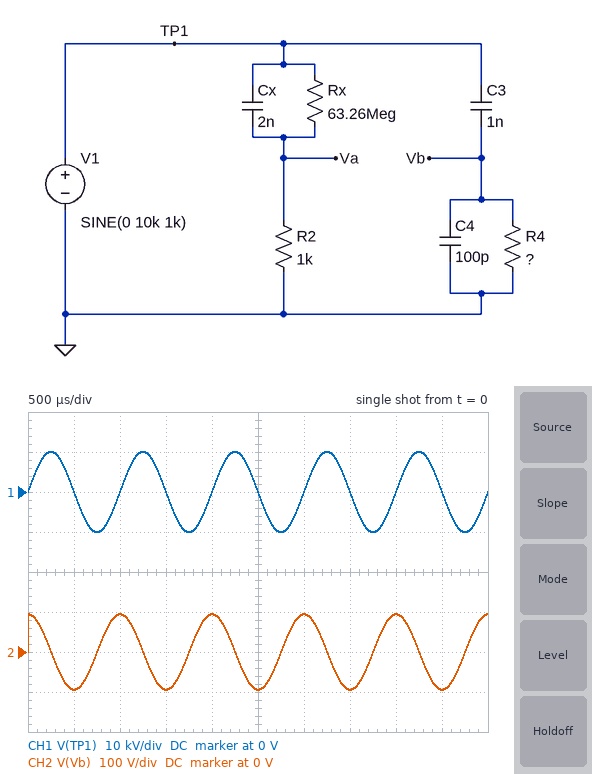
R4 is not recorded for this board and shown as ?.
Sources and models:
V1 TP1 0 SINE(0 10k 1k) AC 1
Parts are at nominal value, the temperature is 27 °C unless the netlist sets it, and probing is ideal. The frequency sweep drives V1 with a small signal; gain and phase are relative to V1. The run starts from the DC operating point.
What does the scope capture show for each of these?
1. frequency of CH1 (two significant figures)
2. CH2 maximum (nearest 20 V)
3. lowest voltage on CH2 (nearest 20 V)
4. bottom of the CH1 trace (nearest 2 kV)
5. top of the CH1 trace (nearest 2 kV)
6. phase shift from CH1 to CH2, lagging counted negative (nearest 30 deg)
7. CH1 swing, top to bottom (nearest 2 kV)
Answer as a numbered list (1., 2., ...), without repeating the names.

1. 1.0 kHz
2. 100 V
3. -100 V
4. -10 kV
5. 10 kV
6. 90 deg
7. 20 kV
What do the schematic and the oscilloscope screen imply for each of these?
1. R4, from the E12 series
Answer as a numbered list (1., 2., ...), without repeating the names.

1. 1.5 kΩ
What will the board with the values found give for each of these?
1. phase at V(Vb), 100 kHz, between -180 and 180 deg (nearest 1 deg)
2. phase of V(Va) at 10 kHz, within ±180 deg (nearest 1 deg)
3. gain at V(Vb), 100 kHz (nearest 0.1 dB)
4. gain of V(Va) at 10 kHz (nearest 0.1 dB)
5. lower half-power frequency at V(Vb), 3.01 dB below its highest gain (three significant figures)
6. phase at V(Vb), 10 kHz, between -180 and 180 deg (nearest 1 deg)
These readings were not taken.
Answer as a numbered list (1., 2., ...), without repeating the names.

1. 44 deg
2. 83 deg
3. -3.7 dB
4. -18.1 dB
5. 96.5 kHz
6. 84 deg
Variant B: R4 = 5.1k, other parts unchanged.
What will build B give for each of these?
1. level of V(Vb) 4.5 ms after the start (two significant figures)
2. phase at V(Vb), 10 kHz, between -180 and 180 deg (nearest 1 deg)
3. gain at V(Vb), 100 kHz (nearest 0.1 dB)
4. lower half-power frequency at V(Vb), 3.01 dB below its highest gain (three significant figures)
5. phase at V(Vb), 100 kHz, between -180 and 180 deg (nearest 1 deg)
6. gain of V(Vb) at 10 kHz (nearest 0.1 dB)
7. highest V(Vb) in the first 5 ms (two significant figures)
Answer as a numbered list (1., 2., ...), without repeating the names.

1. -320 V
2. 71 deg
3. -1.2 dB
4. 28.4 kHz
5. 16 deg
6. -10.4 dB
7. 320 V
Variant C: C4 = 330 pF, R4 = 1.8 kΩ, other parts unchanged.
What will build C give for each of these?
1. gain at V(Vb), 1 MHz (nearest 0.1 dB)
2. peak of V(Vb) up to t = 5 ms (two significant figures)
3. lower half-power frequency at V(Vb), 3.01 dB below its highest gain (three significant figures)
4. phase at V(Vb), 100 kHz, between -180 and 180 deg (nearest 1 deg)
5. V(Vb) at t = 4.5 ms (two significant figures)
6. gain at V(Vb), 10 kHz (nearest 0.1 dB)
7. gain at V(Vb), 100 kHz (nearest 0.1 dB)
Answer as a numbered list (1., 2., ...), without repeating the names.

1. -2.5 dB
2. 110 V
3. 66.5 kHz
4. 34 deg
5. -110 V
6. -19.0 dB
7. -4.1 dB
